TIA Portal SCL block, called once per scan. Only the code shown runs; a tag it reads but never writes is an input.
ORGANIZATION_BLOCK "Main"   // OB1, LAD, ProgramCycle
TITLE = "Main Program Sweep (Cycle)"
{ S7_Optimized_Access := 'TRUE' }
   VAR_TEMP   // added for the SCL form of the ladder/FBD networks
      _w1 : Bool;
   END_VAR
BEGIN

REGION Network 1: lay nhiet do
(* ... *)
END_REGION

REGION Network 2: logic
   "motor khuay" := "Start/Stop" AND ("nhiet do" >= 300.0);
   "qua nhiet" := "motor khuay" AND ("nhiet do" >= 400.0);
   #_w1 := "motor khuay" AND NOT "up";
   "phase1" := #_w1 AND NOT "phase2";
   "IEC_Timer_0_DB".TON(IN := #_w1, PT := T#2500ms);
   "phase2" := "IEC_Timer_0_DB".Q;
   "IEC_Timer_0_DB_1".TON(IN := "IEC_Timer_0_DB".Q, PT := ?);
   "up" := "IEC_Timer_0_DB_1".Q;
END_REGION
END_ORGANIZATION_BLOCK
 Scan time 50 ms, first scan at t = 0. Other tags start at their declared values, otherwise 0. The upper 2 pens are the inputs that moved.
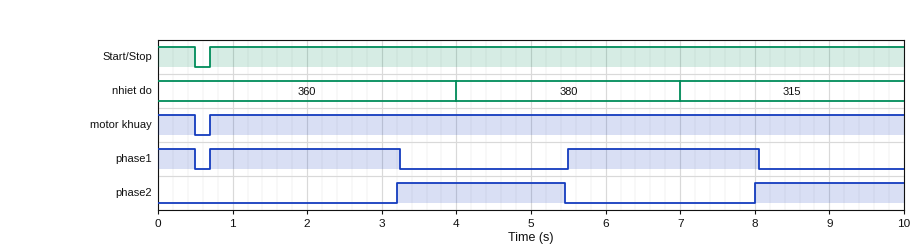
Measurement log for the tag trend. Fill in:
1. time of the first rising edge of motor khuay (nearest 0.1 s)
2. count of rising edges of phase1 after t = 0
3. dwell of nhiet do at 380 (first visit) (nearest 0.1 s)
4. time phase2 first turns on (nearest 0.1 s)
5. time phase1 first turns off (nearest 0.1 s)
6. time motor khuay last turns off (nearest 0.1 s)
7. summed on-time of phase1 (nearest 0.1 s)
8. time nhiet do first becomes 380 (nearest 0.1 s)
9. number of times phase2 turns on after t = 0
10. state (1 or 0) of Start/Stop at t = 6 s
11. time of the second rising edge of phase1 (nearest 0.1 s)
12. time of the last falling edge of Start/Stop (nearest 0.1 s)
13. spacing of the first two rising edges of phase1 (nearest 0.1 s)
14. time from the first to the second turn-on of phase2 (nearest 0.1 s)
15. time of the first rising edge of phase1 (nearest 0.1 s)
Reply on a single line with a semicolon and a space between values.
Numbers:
0.7 s; 2; 3.0 s; 3.2 s; 0.5 s; 0.5 s; 5.6 s; 4.0 s; 2; 1; 5.5 s; 0.5 s; 4.8 s; 4.8 s; 0.7 s
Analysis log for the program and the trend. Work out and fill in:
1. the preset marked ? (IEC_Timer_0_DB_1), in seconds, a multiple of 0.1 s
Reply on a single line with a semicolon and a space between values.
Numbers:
2.2 s
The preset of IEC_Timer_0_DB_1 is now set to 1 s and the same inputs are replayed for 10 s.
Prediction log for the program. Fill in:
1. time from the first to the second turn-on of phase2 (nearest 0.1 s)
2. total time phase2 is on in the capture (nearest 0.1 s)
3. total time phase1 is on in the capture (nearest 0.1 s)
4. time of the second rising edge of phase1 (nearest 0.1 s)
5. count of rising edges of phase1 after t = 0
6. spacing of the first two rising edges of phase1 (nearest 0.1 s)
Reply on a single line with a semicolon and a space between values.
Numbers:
3.6 s; 2.1 s; 7.7 s; 4.3 s; 3; 3.6 s
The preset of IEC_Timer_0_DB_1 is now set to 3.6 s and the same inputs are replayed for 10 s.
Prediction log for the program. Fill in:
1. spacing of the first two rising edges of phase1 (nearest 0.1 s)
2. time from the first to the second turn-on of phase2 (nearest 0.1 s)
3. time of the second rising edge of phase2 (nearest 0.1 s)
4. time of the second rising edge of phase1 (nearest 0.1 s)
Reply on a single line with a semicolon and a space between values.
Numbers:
6.2 s; 6.2 s; 9.4 s; 6.9 s
